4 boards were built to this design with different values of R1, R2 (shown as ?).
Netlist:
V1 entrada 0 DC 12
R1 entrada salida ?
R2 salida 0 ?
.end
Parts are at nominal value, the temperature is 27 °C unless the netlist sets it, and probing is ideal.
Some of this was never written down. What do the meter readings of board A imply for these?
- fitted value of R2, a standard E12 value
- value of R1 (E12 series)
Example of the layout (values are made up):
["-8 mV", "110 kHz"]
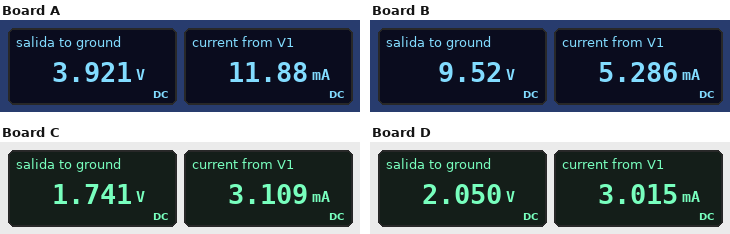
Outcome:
["330 Ω", "680 Ω"]
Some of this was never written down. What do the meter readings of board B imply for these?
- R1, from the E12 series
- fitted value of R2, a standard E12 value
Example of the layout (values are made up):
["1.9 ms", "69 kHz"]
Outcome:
["470 Ω", "1.8 kΩ"]
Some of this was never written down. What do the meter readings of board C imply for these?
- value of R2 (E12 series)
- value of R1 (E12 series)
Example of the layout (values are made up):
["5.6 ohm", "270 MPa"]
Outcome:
["560 Ω", "3.3 kΩ"]
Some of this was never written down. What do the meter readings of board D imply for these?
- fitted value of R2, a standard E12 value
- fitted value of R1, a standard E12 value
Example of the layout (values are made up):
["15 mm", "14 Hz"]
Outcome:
["680 Ω", "3.3 kΩ"]
